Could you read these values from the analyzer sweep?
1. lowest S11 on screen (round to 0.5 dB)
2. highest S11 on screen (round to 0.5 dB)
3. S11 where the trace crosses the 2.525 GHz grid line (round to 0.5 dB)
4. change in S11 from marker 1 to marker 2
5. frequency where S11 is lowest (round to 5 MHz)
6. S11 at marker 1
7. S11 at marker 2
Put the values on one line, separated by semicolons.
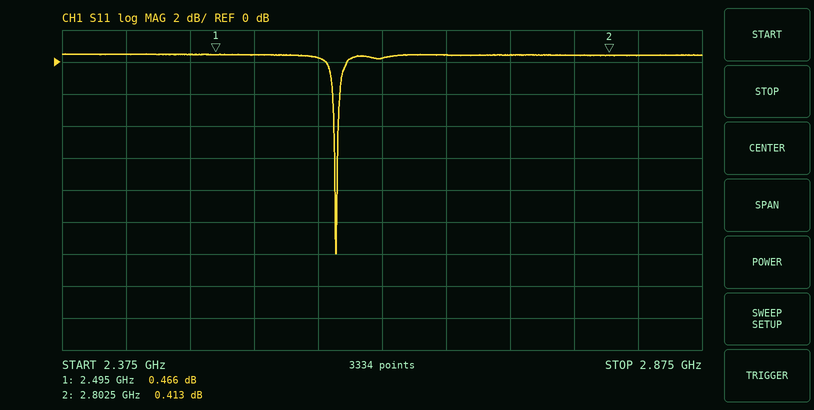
-12.0 dB; 0.5 dB; 0.5 dB; -0.053 dB; 2.590 GHz; 0.466 dB; 0.413 dB
